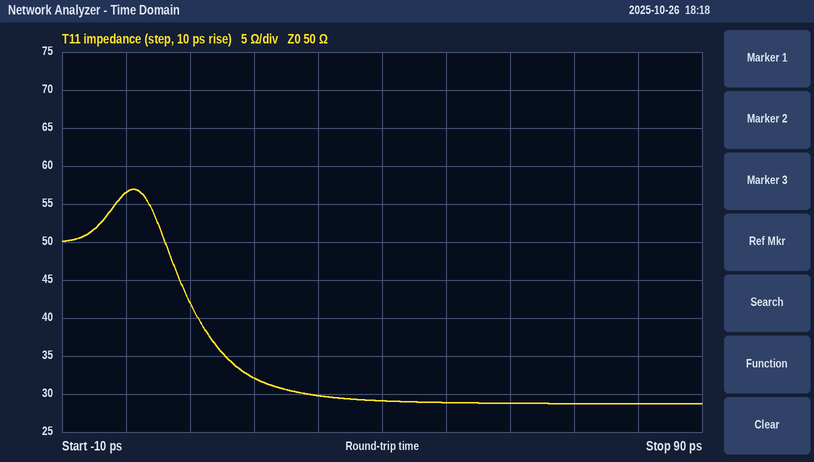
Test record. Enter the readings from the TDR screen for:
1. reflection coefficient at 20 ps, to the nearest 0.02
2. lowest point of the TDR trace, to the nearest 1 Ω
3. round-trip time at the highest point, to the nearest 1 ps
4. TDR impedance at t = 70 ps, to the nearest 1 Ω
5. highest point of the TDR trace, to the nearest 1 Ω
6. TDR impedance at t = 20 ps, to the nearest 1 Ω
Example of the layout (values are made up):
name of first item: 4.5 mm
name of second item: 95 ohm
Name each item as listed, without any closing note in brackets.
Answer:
reflection coefficient at 20 ps, to the nearest 0.02: -0.22
lowest point of the TDR trace, to the nearest 1 Ω: 29 Ω
round-trip time at the highest point, to the nearest 1 ps: 1 ps
TDR impedance at t = 70 ps, to the nearest 1 Ω: 29 Ω
highest point of the TDR trace, to the nearest 1 Ω: 57 Ω
TDR impedance at t = 20 ps, to the nearest 1 Ω: 32 Ω
